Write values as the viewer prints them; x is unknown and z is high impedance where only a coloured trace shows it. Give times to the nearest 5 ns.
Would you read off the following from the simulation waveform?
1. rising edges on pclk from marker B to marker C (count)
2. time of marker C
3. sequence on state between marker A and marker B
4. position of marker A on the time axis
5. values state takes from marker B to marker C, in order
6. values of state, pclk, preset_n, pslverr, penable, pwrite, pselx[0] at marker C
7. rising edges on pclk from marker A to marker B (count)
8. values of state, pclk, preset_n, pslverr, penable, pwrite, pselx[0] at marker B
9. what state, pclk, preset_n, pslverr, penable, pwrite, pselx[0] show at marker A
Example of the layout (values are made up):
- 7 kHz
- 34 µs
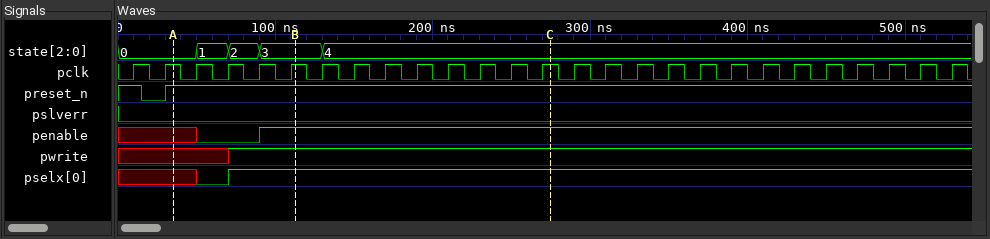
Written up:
- 8
- 275 ns
- 0, 1, 2, 3
- 35 ns
- 3, 4
- state=4, pclk=1, preset_n=1, pslverr=0, penable=1, pwrite=1, pselx[0]=1
- 4
- state=3, pclk=1, preset_n=1, pslverr=0, penable=1, pwrite=1, pselx[0]=1
- state=0, pclk=1, preset_n=1, pslverr=0, penable=x, pwrite=x, pselx[0]=x
